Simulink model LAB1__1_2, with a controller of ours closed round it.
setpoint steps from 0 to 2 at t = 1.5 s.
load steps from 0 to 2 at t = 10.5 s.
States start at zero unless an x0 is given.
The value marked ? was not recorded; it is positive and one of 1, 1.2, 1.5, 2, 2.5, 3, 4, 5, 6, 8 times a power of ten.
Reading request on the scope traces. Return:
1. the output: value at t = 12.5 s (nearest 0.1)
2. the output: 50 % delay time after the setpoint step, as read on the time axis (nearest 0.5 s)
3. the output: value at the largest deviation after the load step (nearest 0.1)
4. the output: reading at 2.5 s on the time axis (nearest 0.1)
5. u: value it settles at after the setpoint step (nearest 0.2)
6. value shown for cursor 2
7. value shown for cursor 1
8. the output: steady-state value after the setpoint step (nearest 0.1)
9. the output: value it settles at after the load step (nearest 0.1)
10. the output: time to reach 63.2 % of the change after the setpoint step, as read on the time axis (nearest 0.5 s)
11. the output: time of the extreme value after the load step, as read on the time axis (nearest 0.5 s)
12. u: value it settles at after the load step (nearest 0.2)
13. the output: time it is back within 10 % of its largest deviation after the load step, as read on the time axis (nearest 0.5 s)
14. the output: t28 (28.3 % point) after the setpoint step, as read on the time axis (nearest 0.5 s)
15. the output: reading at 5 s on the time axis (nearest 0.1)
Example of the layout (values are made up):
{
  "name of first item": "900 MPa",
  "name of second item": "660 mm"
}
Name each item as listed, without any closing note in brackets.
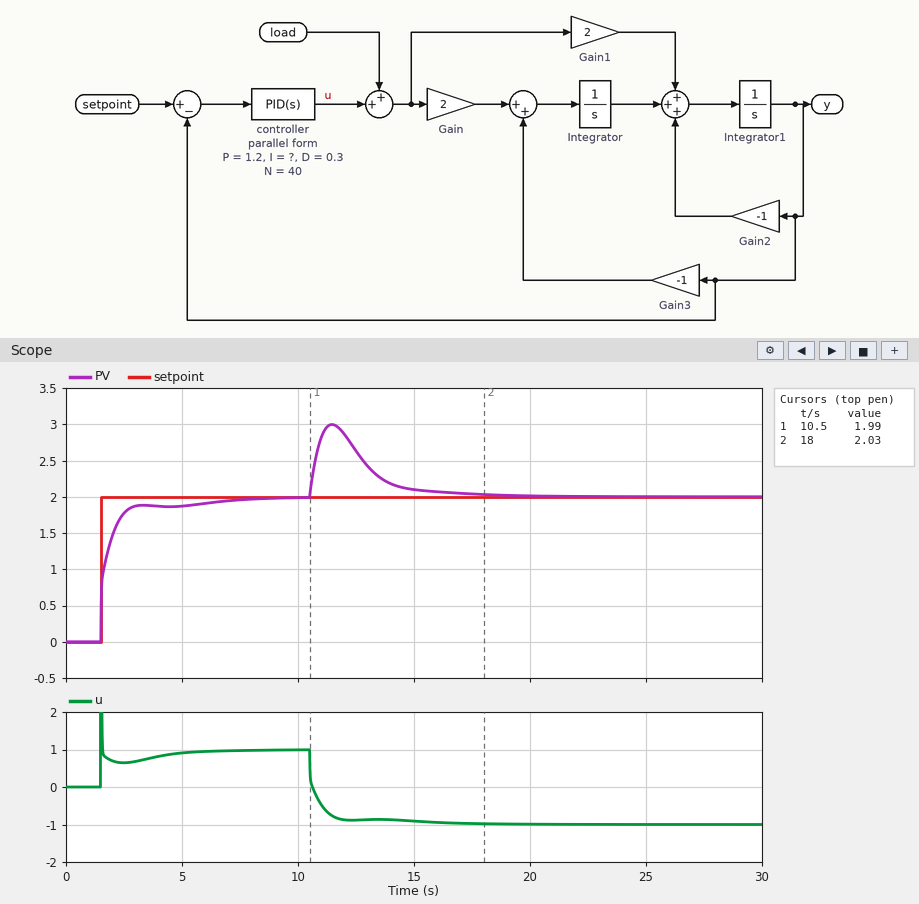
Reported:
{
  "the output: value at t = 12.5 s": "2.6",
  "the output: 50 % delay time after the setpoint step, as read on the time axis": "1.5 s",
  "the output: value at the largest deviation after the load step": "3.0",
  "the output: reading at 2.5 s on the time axis": "1.8",
  "u: value it settles at after the setpoint step": "1.0",
  "value shown for cursor 2": "2.03",
  "value shown for cursor 1": "1.99",
  "the output: steady-state value after the setpoint step": "2.0",
  "the output: value it settles at after the load step": "2.0",
  "the output: time to reach 63.2 % of the change after the setpoint step, as read on the time axis": "2.0 s",
  "the output: time of the extreme value after the load step, as read on the time axis": "11.5 s",
  "u: value it settles at after the load step": "-1.0",
  "the output: time it is back within 10 % of its largest deviation after the load step, as read on the time axis": "15.0 s",
  "the output: t28 (28.3 % point) after the setpoint step, as read on the time axis": "1.5 s",
  "the output: reading at 5 s on the time axis": "1.9"
}
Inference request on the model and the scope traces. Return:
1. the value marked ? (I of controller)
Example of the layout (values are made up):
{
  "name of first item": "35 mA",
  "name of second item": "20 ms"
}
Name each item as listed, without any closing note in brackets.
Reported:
{
  "the value marked ?": "0.8"
}
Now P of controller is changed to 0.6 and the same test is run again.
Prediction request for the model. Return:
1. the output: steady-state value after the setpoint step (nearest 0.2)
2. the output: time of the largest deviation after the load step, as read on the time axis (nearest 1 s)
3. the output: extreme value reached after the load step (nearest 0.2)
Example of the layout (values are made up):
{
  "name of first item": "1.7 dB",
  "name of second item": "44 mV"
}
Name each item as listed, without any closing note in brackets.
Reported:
{
  "the output: steady-state value after the setpoint step": "2.0",
  "the output: time of the largest deviation after the load step, as read on the time axis": "12 s",
  "the output: extreme value reached after the load step": "3.4"
}
